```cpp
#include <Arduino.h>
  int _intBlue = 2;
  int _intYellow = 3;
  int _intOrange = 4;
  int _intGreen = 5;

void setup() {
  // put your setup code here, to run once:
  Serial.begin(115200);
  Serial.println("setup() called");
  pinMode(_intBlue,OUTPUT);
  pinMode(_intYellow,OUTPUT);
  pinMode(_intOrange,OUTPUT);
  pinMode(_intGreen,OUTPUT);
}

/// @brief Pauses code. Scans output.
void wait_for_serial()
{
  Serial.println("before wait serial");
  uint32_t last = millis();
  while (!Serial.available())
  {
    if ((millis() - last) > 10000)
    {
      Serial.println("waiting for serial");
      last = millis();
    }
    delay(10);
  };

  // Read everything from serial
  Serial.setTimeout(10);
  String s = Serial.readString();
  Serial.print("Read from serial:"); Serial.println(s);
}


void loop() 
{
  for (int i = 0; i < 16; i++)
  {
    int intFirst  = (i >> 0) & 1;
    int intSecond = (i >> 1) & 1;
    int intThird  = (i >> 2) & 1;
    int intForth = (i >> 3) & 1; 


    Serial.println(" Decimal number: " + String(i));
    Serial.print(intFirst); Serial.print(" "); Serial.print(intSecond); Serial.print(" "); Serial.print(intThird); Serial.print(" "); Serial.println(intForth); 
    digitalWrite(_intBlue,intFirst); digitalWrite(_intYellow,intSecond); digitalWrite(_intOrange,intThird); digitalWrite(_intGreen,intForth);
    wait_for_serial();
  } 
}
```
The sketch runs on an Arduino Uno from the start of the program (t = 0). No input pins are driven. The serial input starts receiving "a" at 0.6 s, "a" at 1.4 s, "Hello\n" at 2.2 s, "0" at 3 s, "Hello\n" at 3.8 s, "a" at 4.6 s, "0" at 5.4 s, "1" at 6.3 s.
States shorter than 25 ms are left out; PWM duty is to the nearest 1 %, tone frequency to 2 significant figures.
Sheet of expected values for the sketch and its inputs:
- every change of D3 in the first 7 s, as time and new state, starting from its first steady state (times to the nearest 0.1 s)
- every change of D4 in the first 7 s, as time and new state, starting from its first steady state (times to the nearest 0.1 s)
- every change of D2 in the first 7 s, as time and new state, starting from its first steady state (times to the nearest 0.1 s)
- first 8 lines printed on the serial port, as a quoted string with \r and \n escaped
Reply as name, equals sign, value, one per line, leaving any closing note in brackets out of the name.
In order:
every change of D3 in the first 7 s, as time and new state, starting from its first steady state = 0 s low; 1.4 s high; 3 s low; 4.6 s high; 6.3 s low
every change of D4 in the first 7 s, as time and new state, starting from its first steady state = 0 s low; 3 s high; 6.3 s low
every change of D2 in the first 7 s, as time and new state, starting from its first steady state = 0 s low; 0.6 s high; 1.4 s low; 2.2 s high; 3 s low; 3.8 s high; 4.6 s low; 5.4 s high; 6.3 s low
first 8 lines printed on the serial port, as a quoted string with \r and \n escaped = "setup() called\r\n Decimal number: 0\r\n0 0 0 0\r\nbefore wait serial\r\nRead from serial:a\r\n Decimal number: 1\r\n1 0 0 0\r\nbefore wait serial\r\n"
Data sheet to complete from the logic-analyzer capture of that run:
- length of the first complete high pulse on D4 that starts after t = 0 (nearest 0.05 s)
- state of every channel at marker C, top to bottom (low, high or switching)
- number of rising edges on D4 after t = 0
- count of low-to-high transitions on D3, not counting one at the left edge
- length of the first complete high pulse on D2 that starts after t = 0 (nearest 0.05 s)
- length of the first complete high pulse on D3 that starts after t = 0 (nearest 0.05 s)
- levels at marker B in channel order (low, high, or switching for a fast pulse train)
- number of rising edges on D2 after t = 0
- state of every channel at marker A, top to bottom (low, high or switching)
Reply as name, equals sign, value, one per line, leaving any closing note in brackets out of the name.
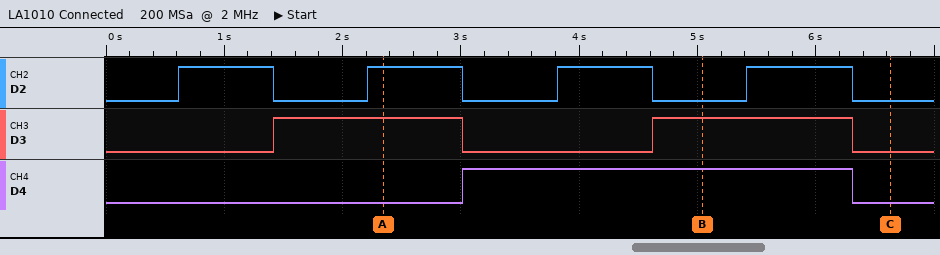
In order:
length of the first complete high pulse on D4 that starts after t = 0 = 3.30 s
state of every channel at marker C, top to bottom = D2 low, D3 low, D4 low
number of rising edges on D4 after t = 0 = 1
count of low-to-high transitions on D3, not counting one at the left edge = 2
length of the first complete high pulse on D2 that starts after t = 0 = 0.80 s
length of the first complete high pulse on D3 that starts after t = 0 = 1.60 s
levels at marker B in channel order = D2 low, D3 high, D4 high
number of rising edges on D2 after t = 0 = 4
state of every channel at marker A, top to bottom = D2 high, D3 high, D4 low
